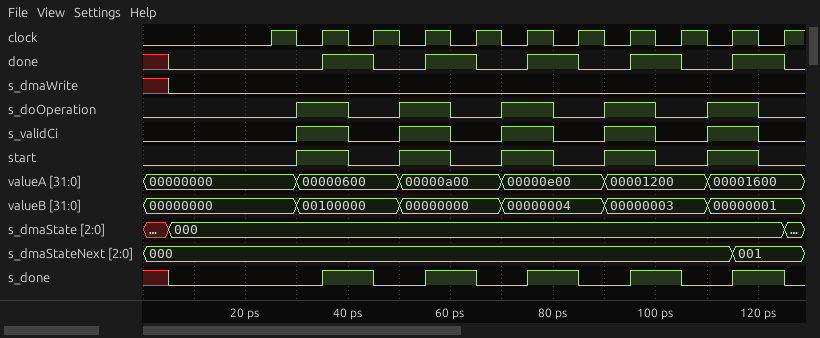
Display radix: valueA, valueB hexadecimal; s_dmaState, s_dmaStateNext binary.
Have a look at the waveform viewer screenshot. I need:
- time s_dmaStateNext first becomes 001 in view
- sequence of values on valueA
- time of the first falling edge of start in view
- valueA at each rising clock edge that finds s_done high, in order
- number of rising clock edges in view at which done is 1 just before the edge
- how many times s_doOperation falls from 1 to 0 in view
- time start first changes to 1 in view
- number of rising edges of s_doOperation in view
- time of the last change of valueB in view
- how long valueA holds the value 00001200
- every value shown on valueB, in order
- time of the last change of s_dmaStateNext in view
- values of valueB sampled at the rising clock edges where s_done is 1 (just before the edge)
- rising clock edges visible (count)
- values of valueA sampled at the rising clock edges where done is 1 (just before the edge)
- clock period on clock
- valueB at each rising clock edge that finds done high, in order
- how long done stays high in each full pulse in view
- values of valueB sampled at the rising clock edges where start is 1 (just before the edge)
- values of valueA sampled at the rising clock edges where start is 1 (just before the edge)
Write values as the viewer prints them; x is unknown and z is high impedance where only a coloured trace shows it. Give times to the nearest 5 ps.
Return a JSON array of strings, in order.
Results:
["115 ps", "00000000, 00000600, 00000a00, 00000e00, 00001200, 00001600", "40 ps", "00000600, 00000a00, 00000e00, 00001200, 00001600", "5", "5", "30 ps", "5", "110 ps", "20 ps", "00000000, 00100000, 00000000, 00000004, 00000003, 00000001", "115 ps", "00100000, 00000000, 00000004, 00000003, 00000001", "11", "00000600, 00000a00, 00000e00, 00001200, 00001600", "10 ps", "00100000, 00000000, 00000004, 00000003, 00000001", "10 ps, 10 ps, 10 ps, 10 ps, 10 ps", "00100000, 00000000, 00000004, 00000003, 00000001", "00000600, 00000a00, 00000e00, 00001200, 00001600"]
